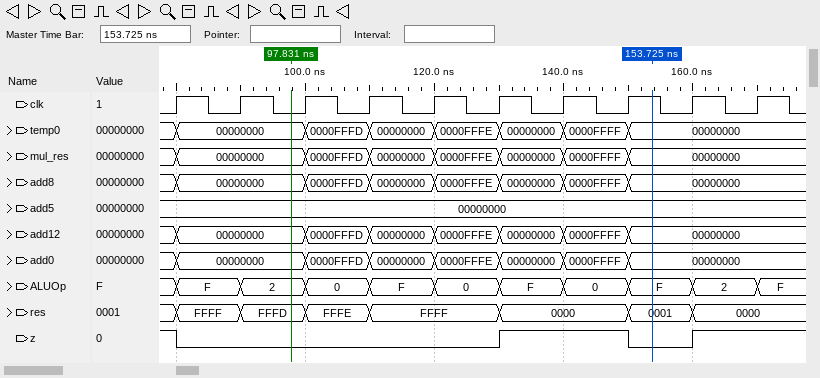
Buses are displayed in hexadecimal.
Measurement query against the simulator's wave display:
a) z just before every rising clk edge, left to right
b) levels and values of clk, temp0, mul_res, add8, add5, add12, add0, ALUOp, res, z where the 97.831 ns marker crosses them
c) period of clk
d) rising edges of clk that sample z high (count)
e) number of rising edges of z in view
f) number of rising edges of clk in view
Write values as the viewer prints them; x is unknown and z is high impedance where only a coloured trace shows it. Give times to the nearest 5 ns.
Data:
1 0 0 0 0 0 1 1 0 1
clk=0, temp0=00000000, mul_res=00000000, add8=00000000, add5=00000000, add12=00000000, add0=00000000, ALUOp=2, res=FFFD, z=0
10 ns
4
2
10
